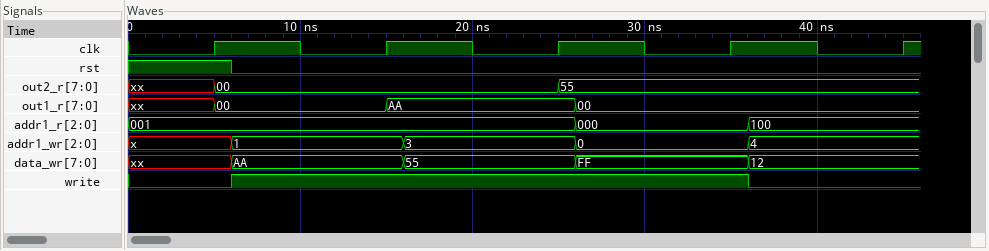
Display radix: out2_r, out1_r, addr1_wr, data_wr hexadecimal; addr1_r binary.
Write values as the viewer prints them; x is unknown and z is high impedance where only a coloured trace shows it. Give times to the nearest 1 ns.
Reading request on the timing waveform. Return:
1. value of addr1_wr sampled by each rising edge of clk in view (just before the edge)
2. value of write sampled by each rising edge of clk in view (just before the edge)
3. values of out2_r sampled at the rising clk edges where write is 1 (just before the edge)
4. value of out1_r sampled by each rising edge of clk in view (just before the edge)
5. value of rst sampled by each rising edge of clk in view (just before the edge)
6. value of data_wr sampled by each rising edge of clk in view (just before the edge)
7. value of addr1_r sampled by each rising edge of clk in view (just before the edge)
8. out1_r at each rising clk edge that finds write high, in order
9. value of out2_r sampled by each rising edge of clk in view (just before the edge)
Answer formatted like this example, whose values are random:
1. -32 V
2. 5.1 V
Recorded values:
1. x, 1, 3, 0, 4
2. 0 1 1 1 0
3. 00, 00, 55
4. xx, 00, AA, 00, 00
5. 1 0 0 0 0
6. xx, AA, 55, FF, 12
7. 001, 001, 001, 000, 100
8. 00, AA, 00
9. xx, 00, 00, 55, 55
